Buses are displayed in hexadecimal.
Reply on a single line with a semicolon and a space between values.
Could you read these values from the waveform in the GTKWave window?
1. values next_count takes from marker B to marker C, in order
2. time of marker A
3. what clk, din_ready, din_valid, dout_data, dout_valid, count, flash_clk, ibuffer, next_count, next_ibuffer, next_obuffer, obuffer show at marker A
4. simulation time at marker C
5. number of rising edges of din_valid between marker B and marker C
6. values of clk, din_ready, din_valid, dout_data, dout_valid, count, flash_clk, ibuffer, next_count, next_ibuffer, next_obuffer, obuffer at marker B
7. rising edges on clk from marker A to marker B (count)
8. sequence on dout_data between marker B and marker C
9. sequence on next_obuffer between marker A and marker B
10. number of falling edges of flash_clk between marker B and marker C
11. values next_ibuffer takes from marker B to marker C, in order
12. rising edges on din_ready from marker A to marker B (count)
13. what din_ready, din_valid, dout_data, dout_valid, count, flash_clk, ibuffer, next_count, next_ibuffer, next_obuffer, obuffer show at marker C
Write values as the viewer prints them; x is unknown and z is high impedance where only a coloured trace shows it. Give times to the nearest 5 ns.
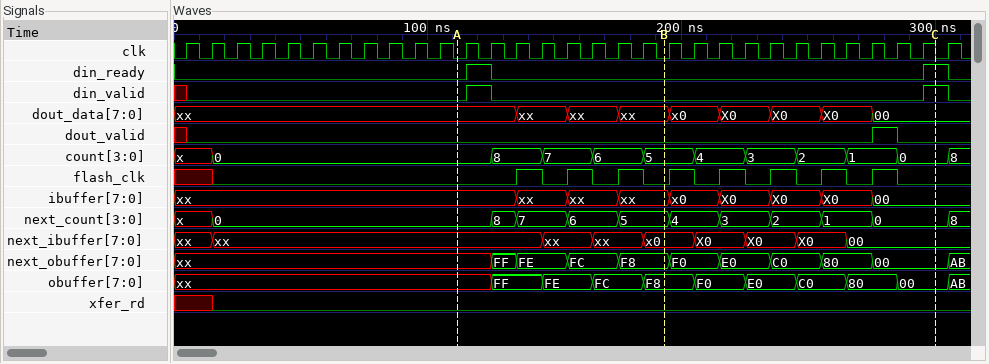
5, 4, 3, 2, 1, 0; 110 ns; clk=0, din_ready=0, din_valid=0, dout_data=xx, dout_valid=0, count=0, flash_clk=0, ibuffer=xx, next_count=0, next_ibuffer=xx, next_obuffer=xx, obuffer=xx; 300 ns; 1; clk=0, din_ready=0, din_valid=0, dout_data=xx, dout_valid=0, count=5, flash_clk=0, ibuffer=xx, next_count=5, next_ibuffer=x0, next_obuffer=F8, obuffer=F8; 8; xx, x0, X0, X0, X0, 00; xx, FF, FE, FC, F8; 5; x0, X0, X0, X0, 00; 1; din_ready=1, din_valid=1, dout_data=00, dout_valid=0, count=0, flash_clk=0, ibuffer=00, next_count=0, next_ibuffer=00, next_obuffer=00, obuffer=00
